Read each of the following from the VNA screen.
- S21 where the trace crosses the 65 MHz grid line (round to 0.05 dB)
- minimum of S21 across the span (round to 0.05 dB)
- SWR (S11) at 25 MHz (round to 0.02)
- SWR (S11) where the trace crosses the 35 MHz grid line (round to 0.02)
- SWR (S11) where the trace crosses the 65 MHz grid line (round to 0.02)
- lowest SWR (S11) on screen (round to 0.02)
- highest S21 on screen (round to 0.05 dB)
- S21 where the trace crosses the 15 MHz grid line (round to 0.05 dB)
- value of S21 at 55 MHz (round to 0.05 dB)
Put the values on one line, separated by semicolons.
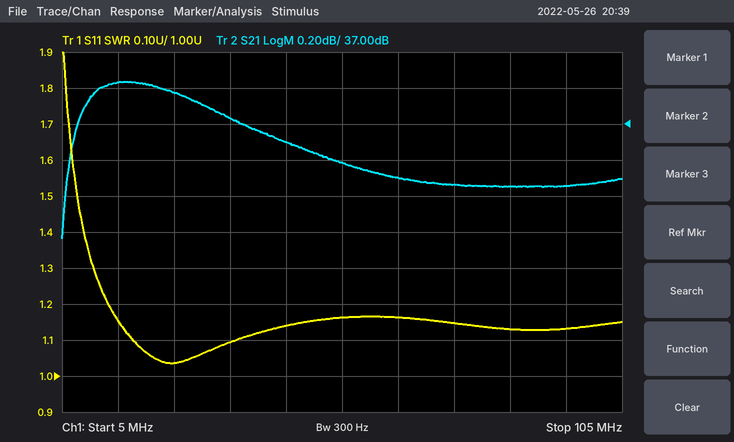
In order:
36.70 dB; 36.35 dB; 1.04; 1.10; 1.16; 1.04; 37.25 dB; 37.25 dB; 36.80 dB
